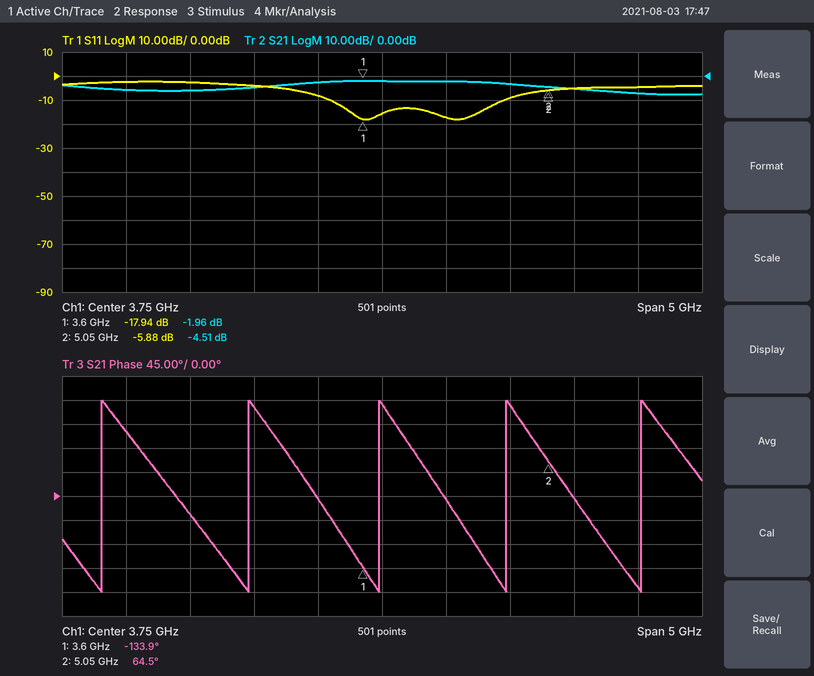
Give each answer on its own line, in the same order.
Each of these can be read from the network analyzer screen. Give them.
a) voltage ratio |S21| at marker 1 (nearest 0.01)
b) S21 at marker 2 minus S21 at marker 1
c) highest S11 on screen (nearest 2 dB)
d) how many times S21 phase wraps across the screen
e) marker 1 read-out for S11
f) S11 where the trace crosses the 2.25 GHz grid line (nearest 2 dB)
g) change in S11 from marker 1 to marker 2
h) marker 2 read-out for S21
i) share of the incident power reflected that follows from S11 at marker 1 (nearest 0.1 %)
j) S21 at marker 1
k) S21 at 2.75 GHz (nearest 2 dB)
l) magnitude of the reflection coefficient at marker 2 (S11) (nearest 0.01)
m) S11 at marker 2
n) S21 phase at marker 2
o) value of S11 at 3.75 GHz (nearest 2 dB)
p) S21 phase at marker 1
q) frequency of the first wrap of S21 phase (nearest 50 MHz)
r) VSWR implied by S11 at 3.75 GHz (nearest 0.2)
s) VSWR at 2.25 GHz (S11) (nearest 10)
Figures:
0.80
-2.55 dB
-2 dB
5
-17.94 dB
-2 dB
12.06 dB
-4.51 dB
1.6 %
-1.96 dB
-4 dB
0.51
-5.88 dB
64.5°
-16 dB
-133.9°
1.55 GHz
1.4
10
